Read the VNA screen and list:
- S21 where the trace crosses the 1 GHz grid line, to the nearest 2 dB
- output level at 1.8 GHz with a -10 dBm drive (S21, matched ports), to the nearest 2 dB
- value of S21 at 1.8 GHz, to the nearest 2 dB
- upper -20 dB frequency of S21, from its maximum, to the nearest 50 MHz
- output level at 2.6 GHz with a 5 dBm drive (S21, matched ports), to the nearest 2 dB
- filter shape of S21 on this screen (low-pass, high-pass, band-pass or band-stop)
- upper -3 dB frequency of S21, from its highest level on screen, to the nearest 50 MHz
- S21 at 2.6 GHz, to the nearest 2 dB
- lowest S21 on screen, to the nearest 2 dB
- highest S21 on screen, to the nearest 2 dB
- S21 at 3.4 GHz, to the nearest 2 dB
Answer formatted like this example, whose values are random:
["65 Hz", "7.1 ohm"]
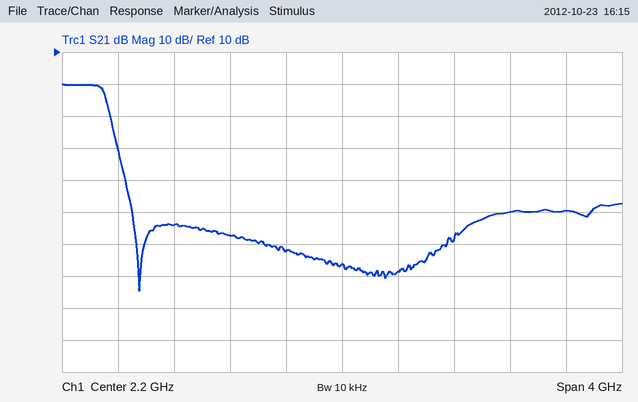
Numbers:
["-44 dB", "-62 dBm", "-52 dB", "600 MHz", "-54 dBm", "low-pass", "500 MHz", "-58 dB", "-64 dB", "0 dB", "-40 dB"]
